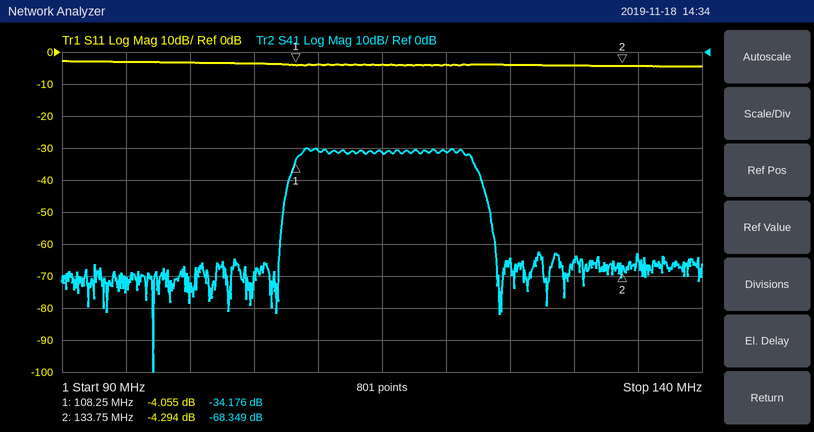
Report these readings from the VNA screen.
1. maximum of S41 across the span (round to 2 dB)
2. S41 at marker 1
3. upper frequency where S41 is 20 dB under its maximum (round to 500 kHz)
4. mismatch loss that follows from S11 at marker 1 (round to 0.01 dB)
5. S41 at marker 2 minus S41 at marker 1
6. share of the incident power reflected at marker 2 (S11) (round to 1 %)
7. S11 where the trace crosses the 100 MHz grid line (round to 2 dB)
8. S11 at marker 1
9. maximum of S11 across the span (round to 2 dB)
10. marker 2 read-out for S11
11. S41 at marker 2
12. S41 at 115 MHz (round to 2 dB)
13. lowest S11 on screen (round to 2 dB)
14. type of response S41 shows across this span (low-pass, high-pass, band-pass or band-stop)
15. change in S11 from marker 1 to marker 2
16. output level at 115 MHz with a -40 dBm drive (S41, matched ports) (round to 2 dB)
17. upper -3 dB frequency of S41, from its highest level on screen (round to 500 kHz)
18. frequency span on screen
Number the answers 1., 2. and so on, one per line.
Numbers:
1. -30 dB
2. -34.176 dB
3. 123.5 MHz
4. 2.17 dB
5. -34.173 dB
6. 37 %
7. -4 dB
8. -4.055 dB
9. -2 dB
10. -4.294 dB
11. -68.349 dB
12. -32 dB
13. -4 dB
14. band-pass
15. -0.239 dB
16. -72 dBm
17. 122.0 MHz
18. 50 MHz
